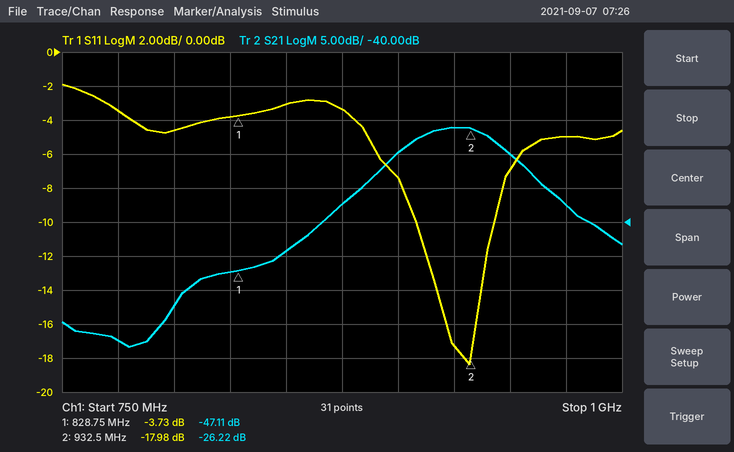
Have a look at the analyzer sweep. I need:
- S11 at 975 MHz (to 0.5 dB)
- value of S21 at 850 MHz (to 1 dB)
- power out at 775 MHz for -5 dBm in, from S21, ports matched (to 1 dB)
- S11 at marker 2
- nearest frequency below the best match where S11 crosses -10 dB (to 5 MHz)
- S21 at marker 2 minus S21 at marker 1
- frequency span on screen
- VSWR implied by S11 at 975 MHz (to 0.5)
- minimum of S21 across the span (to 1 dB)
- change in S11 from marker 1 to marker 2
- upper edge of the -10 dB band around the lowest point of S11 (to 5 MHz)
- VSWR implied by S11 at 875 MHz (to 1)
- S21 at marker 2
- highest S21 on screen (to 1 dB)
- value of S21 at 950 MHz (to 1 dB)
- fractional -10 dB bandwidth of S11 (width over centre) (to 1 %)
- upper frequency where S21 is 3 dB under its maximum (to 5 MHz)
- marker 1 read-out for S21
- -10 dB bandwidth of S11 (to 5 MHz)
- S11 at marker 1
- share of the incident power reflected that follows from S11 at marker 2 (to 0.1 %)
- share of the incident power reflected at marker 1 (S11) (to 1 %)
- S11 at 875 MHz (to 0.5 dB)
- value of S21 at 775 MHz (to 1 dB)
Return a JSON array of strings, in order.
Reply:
["-5.0 dB", "-44 dB", "-62 dBm", "-17.98 dB", "910 MHz", "20.89 dB", "250 MHz", "3.5", "-58 dB", "-14.25 dB", "945 MHz", "5", "-26.22 dB", "-26 dB", "-30 dB", "4 %", "945 MHz", "-47.11 dB", "35 MHz", "-3.73 dB", "1.6 %", "42 %", "-3.5 dB", "-57 dB"]
